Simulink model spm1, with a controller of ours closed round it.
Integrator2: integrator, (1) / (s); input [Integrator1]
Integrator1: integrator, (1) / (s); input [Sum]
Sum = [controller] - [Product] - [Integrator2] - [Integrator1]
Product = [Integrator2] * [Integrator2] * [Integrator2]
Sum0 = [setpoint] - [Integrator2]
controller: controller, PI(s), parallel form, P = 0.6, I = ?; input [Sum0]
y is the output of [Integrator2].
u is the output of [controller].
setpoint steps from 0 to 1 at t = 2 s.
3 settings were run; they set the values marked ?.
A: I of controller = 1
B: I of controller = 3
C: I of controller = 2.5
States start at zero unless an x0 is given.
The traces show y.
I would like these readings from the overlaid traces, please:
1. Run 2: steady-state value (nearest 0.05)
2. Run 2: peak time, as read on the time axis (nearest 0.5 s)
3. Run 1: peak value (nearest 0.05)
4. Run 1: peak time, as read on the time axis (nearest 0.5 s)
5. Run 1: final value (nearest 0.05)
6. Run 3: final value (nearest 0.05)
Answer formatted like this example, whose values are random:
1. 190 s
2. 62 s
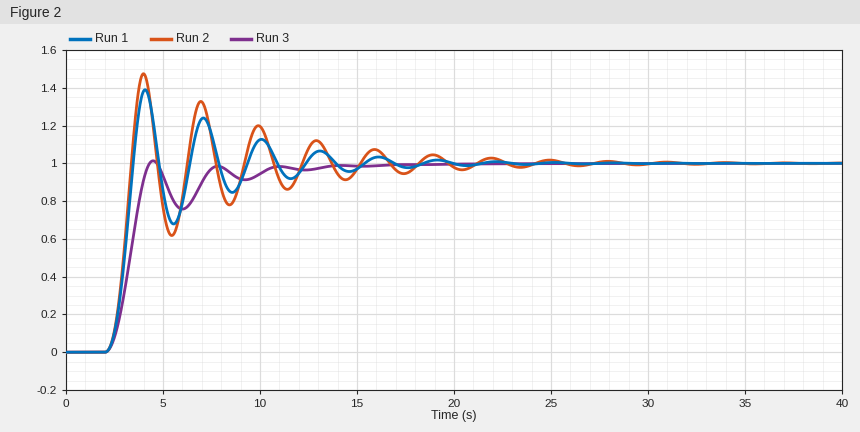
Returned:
1. 1.00
2. 4.0 s
3. 1.40
4. 4.0 s
5. 1.00
6. 1.00
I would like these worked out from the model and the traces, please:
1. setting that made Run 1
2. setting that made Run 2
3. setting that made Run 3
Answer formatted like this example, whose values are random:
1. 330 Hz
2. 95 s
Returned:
1. C
2. B
3. A
